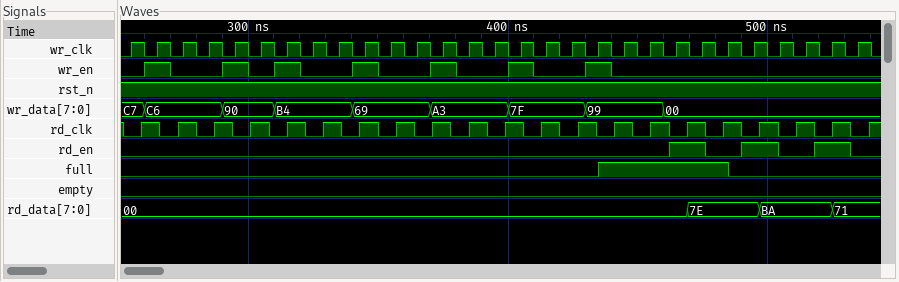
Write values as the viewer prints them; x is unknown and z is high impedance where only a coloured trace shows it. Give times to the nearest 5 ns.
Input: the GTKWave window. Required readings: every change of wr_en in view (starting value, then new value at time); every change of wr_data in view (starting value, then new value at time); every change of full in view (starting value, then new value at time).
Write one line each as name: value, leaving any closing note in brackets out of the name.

every change of wr_en in view: 0, 1 at 260 ns, 0 at 270 ns, 1 at 290 ns, 0 at 300 ns, 1 at 310 ns, 0 at 320 ns, 1 at 340 ns, 0 at 350 ns, 1 at 370 ns, 0 at 380 ns, 1 at 400 ns, 0 at 410 ns, 1 at 430 ns, 0 at 440 ns
every change of wr_data in view: C7, C6 at 260 ns, 90 at 290 ns, B4 at 310 ns, 69 at 340 ns, A3 at 370 ns, 7F at 400 ns, 99 at 430 ns, 00 at 460 ns
every change of full in view: 0, 1 at 435 ns, 0 at 485 ns
